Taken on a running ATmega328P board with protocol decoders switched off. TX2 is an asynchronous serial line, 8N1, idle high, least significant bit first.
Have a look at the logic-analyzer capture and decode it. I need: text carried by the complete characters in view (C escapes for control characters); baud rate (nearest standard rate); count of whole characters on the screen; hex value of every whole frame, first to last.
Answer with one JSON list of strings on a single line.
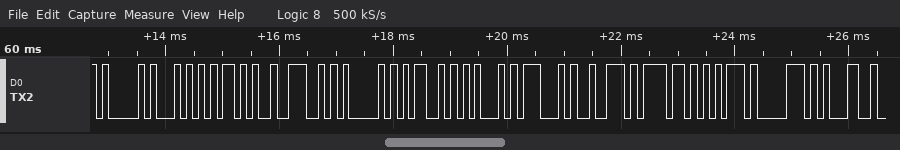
["\"AT+NAMEGroup1\"", "9600 baud", "13", "0x41 0x54 0x2B 0x4E 0x41 0x4D 0x45 0x47 0x72 0x6F 0x75 0x70 0x31"]
